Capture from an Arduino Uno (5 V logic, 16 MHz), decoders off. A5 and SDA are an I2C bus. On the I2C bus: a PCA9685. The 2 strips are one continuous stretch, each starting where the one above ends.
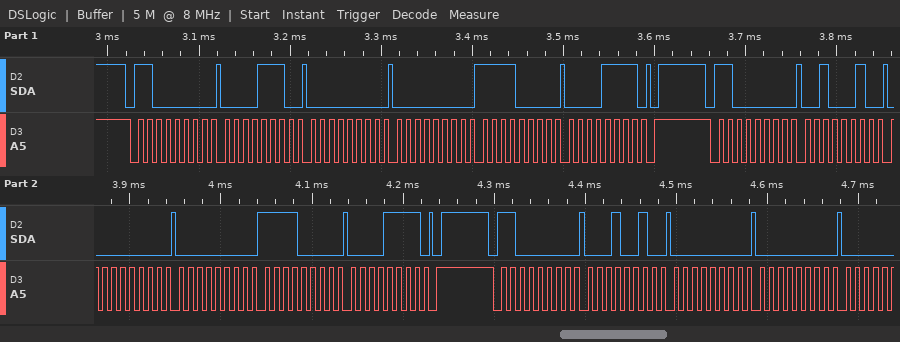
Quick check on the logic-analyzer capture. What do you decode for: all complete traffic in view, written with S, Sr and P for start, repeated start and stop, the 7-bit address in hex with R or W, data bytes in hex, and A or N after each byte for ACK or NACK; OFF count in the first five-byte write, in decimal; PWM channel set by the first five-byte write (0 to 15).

S 60W A 0E A 00 A 00 A F0 A 0F A P S 60W A 22 A 00 A 00 A F0 A 0F A P S 60W A 12 A 00 A 00 A
4080
2
